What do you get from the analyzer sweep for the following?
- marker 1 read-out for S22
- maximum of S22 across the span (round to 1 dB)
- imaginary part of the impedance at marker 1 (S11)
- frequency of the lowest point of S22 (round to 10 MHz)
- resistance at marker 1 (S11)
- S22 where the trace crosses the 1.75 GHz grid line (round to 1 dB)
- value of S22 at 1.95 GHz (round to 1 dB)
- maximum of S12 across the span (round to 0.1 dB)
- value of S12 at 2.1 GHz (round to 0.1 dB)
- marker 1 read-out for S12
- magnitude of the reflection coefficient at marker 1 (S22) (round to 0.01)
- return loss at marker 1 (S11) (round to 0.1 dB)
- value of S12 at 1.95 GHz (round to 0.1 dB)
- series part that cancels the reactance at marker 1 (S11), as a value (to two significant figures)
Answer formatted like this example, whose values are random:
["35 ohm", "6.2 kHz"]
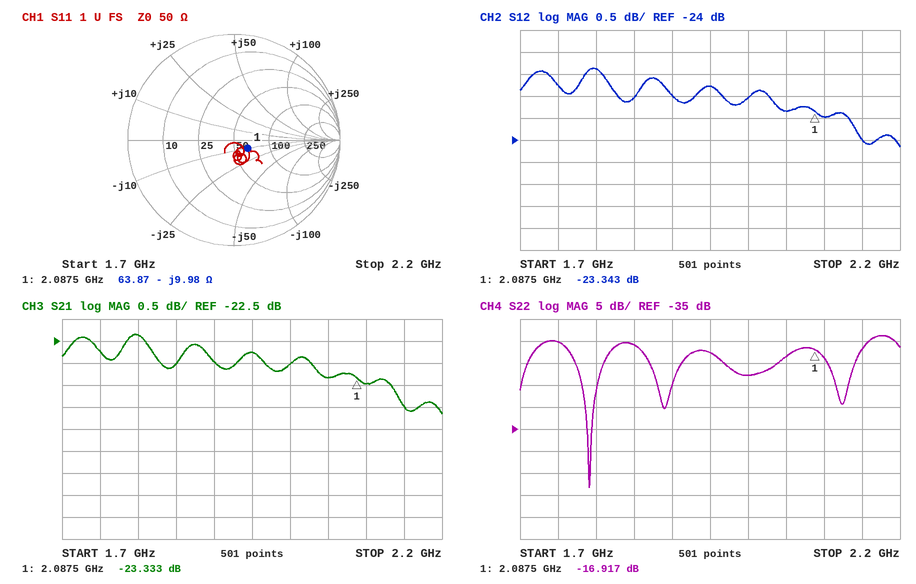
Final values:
["-16.917 dB", "-14 dB", "-9.98 Ω", "1.79 GHz", "63.87 Ω", "-15 dB", "-18 dB", "-22.4 dB", "-23.5 dB", "-23.343 dB", "0.14", "16.5 dB", "-22.8 dB", "760 pH"]
